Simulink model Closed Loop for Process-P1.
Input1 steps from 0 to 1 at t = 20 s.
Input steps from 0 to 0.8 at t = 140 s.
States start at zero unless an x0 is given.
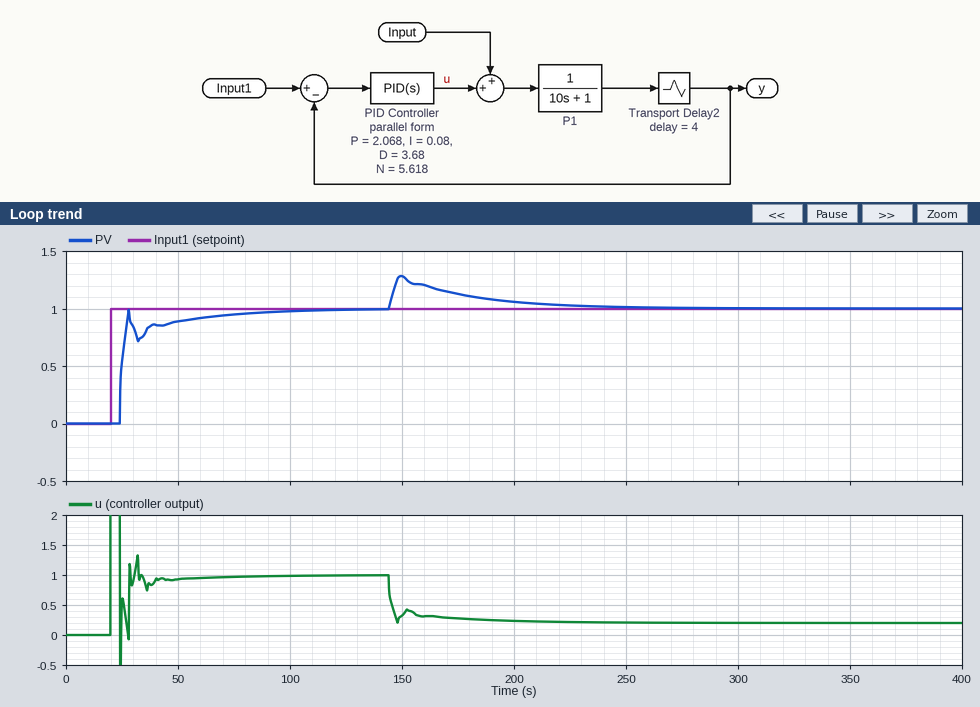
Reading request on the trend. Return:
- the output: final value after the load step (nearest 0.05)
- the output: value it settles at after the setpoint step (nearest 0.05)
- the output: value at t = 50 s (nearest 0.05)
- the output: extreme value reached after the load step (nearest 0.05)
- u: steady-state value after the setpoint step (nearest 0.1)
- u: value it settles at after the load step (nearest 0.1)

1.00
1.00
0.90
1.30
1.0
0.2
